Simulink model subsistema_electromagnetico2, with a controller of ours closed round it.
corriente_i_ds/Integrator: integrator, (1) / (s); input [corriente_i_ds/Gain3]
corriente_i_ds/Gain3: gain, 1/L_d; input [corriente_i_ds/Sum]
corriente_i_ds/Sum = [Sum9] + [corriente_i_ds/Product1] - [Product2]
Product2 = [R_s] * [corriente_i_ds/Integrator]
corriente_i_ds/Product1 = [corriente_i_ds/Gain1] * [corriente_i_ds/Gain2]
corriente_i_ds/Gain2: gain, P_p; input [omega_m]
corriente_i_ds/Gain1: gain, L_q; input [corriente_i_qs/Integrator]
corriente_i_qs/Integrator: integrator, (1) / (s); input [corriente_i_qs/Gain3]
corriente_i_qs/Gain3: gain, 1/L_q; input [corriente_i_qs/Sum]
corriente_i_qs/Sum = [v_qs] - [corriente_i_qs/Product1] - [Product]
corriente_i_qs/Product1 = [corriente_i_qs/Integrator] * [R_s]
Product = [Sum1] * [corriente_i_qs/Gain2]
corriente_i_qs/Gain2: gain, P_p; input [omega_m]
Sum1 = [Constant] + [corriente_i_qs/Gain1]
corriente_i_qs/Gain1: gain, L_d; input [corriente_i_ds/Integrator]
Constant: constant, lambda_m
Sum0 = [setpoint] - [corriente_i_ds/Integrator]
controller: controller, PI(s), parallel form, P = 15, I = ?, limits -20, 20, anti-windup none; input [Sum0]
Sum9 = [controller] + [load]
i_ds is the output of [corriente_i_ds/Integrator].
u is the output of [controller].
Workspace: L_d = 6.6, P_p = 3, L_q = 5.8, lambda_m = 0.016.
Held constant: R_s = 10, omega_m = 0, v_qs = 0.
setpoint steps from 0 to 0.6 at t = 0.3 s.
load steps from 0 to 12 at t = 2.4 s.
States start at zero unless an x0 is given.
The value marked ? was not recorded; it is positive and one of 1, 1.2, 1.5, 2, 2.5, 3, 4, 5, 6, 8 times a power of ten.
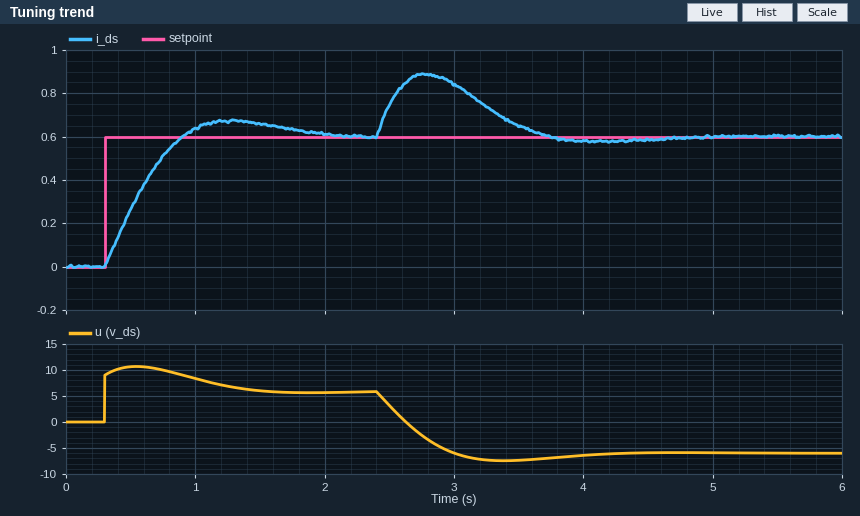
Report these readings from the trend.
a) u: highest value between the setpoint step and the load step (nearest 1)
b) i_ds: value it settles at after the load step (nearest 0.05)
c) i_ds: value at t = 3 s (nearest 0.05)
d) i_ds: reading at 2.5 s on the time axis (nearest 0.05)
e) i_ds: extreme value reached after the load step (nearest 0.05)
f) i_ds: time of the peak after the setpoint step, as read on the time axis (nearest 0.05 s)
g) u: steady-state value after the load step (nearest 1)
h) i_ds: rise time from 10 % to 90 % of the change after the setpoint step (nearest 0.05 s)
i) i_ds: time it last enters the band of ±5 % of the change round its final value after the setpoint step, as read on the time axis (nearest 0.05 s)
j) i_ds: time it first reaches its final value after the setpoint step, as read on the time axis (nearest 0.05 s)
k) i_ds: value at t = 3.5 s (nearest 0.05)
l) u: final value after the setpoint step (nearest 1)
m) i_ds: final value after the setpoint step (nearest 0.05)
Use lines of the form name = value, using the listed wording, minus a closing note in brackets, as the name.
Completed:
u: highest value between the setpoint step and the load step = 11
i_ds: value it settles at after the load step = 0.60
i_ds: value at t = 3 s = 0.85
i_ds: reading at 2.5 s on the time axis = 0.75
i_ds: extreme value reached after the load step = 0.90
i_ds: time of the peak after the setpoint step, as read on the time axis = 1.30 s
u: steady-state value after the load step = -6
i_ds: rise time from 10 % to 90 % of the change after the setpoint step = 0.45 s
i_ds: time it last enters the band of ±5 % of the change round its final value after the setpoint step, as read on the time axis = 1.80 s
i_ds: time it first reaches its final value after the setpoint step, as read on the time axis = 0.90 s
i_ds: value at t = 3.5 s = 0.65
u: final value after the setpoint step = 6
i_ds: final value after the setpoint step = 0.60
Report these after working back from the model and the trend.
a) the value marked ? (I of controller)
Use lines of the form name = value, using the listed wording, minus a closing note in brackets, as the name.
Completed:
the value marked ? = 60
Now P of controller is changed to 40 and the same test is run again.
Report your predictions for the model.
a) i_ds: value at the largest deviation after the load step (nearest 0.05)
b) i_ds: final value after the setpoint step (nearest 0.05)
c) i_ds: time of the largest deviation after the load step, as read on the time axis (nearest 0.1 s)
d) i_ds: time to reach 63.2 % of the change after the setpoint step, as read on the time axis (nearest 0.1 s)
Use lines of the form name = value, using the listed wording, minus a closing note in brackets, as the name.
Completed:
i_ds: value at the largest deviation after the load step = 0.80
i_ds: final value after the setpoint step = 0.60
i_ds: time of the largest deviation after the load step, as read on the time axis = 2.7 s
i_ds: time to reach 63.2 % of the change after the setpoint step, as read on the time axis = 0.5 s
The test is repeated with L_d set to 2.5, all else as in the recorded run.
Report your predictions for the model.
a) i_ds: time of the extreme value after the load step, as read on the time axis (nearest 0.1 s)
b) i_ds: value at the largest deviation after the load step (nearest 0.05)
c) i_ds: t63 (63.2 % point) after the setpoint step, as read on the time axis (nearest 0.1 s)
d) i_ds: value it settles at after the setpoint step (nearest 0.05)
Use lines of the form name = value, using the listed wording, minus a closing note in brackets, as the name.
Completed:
i_ds: time of the extreme value after the load step, as read on the time axis = 2.6 s
i_ds: value at the largest deviation after the load step = 0.95
i_ds: t63 (63.2 % point) after the setpoint step, as read on the time axis = 0.5 s
i_ds: value it settles at after the setpoint step = 0.60
